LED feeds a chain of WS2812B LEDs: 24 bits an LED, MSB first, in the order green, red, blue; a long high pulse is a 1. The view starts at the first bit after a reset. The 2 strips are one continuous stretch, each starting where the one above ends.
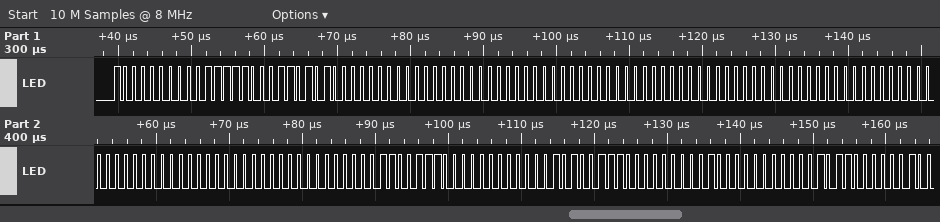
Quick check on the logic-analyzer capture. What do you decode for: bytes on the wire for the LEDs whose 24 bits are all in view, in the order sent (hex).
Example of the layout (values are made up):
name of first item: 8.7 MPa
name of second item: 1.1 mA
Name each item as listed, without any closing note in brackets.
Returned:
bytes on the wire for the LEDs whose 24 bits are all in view, in the order sent: 80 3E 35 00 00 00 00 00 00 00 00 00 00 00 00 67 00 0A 70 04 00
